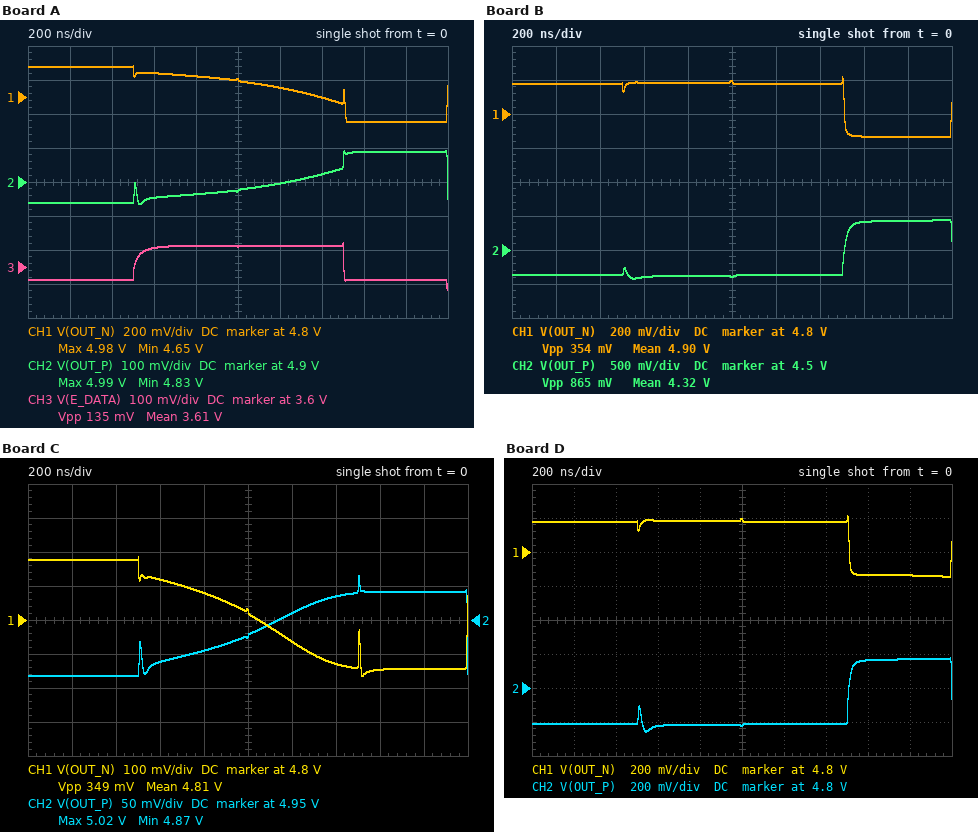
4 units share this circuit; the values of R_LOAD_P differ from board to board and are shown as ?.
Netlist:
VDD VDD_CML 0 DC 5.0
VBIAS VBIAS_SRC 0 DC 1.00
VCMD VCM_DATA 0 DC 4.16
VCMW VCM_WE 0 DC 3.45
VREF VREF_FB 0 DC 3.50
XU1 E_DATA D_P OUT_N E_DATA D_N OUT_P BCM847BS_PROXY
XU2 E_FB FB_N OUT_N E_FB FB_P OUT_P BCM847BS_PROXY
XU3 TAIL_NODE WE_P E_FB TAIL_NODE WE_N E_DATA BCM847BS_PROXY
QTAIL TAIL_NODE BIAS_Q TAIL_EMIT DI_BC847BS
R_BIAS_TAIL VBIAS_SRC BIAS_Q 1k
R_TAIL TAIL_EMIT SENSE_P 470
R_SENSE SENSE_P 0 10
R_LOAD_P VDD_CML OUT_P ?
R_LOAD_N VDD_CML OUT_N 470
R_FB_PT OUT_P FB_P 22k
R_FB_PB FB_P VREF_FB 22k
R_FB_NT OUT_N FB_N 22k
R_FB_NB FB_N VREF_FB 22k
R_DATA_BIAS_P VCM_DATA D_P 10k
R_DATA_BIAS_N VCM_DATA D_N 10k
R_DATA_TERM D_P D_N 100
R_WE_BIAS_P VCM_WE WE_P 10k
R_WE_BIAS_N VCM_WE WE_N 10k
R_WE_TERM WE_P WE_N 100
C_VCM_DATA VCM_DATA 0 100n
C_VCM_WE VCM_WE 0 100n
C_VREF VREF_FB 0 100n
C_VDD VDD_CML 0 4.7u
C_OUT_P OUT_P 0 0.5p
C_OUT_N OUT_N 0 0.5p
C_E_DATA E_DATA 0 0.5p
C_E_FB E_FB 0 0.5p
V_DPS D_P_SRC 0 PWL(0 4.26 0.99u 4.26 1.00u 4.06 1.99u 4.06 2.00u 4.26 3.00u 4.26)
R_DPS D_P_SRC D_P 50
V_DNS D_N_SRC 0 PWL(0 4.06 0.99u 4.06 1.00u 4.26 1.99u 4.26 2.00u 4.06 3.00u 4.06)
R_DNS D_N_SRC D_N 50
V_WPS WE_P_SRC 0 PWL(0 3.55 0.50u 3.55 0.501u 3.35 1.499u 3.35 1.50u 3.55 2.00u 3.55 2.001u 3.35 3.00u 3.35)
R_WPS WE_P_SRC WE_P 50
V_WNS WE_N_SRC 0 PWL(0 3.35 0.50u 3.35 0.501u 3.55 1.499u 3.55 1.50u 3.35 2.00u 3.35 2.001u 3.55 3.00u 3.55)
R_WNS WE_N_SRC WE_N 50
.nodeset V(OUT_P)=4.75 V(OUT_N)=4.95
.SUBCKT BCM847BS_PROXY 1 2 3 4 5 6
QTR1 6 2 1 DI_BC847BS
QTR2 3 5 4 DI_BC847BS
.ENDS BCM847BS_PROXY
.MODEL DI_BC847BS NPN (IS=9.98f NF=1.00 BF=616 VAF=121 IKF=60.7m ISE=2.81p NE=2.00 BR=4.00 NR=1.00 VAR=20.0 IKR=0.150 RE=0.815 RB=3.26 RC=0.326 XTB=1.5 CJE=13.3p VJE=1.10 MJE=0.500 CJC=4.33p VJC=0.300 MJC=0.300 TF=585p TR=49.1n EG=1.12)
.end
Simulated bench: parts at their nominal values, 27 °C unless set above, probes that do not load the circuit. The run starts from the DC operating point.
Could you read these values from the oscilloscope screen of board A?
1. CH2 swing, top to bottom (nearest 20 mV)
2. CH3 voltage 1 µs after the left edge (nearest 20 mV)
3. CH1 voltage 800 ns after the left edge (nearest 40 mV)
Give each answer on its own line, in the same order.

160 mV
3.66 V
4.92 V
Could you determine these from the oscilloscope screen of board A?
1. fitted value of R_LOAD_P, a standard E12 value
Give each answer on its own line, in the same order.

220 Ω
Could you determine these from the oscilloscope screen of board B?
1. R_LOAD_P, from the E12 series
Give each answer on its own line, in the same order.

1.2 kΩ
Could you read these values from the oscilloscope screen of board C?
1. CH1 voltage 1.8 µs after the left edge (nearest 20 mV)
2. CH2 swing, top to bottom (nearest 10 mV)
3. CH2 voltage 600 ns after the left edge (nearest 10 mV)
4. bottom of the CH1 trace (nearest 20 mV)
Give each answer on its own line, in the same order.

4.66 V
150 mV
4.89 V
4.64 V
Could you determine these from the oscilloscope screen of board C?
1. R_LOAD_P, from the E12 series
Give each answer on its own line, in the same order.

180 Ω
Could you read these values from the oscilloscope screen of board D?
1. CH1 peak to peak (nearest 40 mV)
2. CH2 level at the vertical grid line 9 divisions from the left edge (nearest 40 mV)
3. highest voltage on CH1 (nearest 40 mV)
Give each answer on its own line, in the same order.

360 mV
4.96 V
5.00 V
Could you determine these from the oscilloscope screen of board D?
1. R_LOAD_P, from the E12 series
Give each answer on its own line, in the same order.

560 Ω
